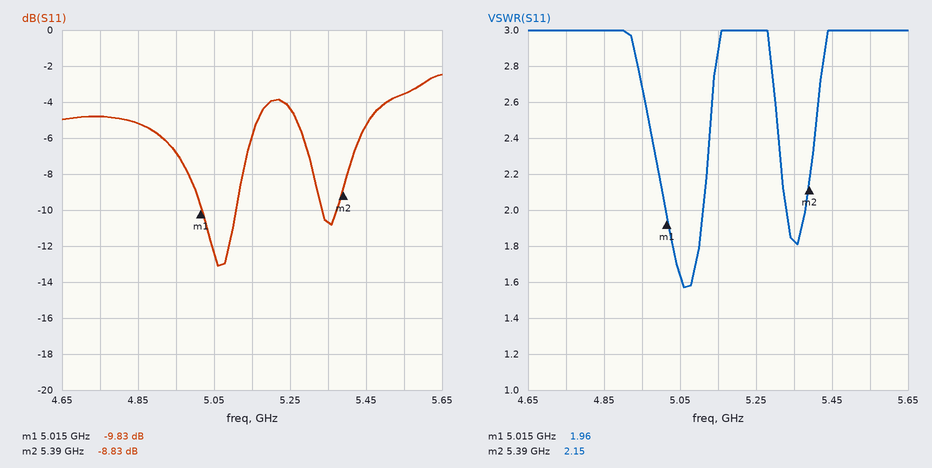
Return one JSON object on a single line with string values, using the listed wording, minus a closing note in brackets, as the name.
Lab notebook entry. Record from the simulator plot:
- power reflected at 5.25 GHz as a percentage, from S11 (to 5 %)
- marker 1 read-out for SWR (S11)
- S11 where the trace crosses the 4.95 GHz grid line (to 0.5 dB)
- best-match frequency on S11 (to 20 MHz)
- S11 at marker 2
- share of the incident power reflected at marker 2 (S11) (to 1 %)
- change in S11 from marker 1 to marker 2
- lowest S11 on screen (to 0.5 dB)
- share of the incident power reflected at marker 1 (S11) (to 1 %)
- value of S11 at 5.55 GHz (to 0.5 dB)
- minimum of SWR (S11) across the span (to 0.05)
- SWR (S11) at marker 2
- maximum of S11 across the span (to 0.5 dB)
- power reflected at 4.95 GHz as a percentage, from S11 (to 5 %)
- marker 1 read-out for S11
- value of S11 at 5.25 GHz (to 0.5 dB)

{"power reflected at 5.25 GHz as a percentage, from S11": "35 %", "marker 1 read-out for SWR": "1.96", "S11 where the trace crosses the 4.95 GHz grid line": "-7.0 dB", "best-match frequency on S11": "5.06 GHz", "S11 at marker 2": "-8.83 dB", "share of the incident power reflected at marker 2 (S11)": "13 %", "change in S11 from marker 1 to marker 2": "1.00 dB", "lowest S11 on screen": "-13.0 dB", "share of the incident power reflected at marker 1 (S11)": "10 %", "value of S11 at 5.55 GHz": "-3.5 dB", "minimum of SWR (S11) across the span": "1.55", "SWR (S11) at marker 2": "2.15", "maximum of S11 across the span": "-2.5 dB", "power reflected at 4.95 GHz as a percentage, from S11": "20 %", "marker 1 read-out for S11": "-9.83 dB", "value of S11 at 5.25 GHz": "-4.5 dB"}
